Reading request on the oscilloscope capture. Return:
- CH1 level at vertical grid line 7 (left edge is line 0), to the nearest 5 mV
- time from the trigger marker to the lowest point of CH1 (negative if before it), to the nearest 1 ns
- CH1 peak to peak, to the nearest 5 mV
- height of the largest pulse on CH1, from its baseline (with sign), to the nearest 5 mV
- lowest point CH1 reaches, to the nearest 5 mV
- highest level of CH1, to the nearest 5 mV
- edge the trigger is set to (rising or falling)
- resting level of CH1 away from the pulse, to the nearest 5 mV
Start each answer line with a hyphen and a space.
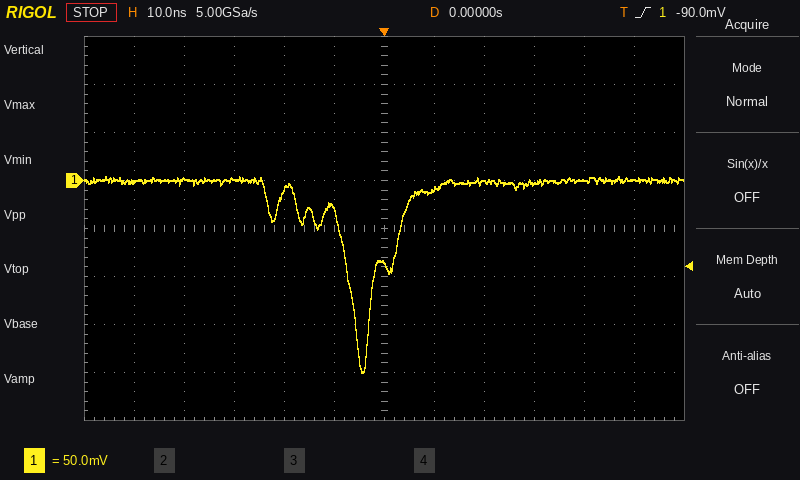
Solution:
- -10 mV
- -4 ns
- 205 mV
- -200 mV
- -200 mV
- 5 mV
- rising
- 0 mV
